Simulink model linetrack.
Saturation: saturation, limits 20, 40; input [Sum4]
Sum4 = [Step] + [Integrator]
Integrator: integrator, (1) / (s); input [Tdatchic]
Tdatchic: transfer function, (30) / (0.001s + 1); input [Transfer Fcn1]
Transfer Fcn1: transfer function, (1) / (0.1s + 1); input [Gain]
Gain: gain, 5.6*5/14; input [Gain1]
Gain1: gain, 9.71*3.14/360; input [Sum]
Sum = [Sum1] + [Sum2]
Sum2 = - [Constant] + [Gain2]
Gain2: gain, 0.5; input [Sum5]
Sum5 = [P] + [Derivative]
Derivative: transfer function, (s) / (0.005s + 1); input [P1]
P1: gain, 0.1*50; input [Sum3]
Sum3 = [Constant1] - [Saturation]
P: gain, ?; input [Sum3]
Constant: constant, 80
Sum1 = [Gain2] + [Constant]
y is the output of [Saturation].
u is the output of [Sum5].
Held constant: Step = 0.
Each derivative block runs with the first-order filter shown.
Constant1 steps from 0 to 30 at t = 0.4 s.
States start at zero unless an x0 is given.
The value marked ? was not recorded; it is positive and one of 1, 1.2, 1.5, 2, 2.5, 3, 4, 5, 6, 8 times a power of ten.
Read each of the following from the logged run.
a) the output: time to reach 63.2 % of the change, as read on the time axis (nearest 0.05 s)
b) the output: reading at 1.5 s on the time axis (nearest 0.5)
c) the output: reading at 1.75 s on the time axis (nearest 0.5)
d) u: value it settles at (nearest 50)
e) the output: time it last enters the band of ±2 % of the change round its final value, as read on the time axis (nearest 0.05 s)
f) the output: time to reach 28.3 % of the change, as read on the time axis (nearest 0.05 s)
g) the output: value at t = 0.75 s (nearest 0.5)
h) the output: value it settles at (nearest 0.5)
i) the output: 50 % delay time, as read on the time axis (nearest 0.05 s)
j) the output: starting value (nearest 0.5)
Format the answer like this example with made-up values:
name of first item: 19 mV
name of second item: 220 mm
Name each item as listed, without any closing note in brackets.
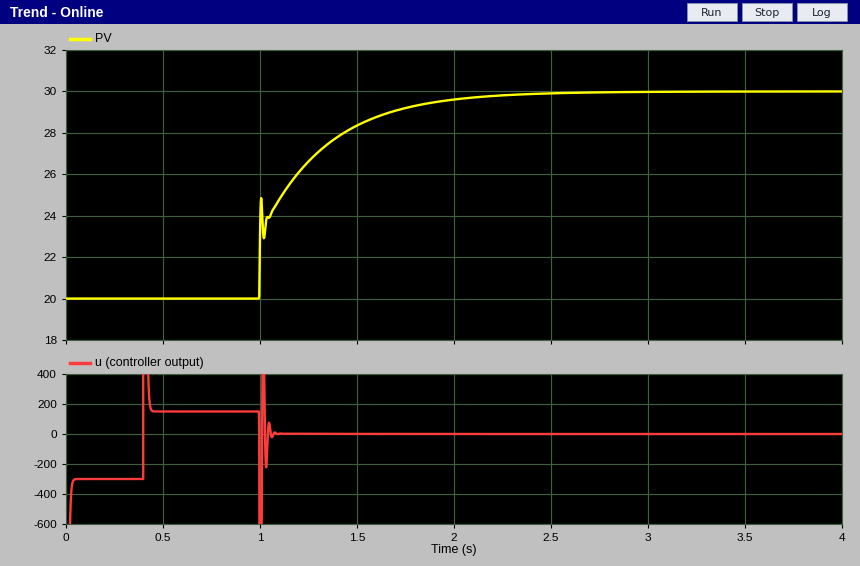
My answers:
the output: time to reach 63.2 % of the change, as read on the time axis: 1.20 s
the output: reading at 1.5 s on the time axis: 28.5
the output: reading at 1.75 s on the time axis: 29.0
u: value it settles at: 0
the output: time it last enters the band of ±2 % of the change round its final value, as read on the time axis: 2.25 s
the output: time to reach 28.3 % of the change, as read on the time axis: 1.00 s
the output: value at t = 0.75 s: 20.0
the output: value it settles at: 30.0
the output: 50 % delay time, as read on the time axis: 1.10 s
the output: starting value: 20.0
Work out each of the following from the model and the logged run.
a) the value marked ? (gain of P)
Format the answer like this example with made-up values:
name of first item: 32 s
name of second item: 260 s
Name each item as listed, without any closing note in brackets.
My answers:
the value marked ?: 15
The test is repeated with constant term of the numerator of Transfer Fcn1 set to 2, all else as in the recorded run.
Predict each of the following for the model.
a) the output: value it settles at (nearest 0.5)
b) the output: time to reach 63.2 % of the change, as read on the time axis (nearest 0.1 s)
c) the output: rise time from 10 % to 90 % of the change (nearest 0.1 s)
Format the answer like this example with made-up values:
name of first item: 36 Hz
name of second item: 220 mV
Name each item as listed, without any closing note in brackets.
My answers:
the output: value it settles at: 30.0
the output: time to reach 63.2 % of the change, as read on the time axis: 1.0 s
the output: rise time from 10 % to 90 % of the change: 0.7 s
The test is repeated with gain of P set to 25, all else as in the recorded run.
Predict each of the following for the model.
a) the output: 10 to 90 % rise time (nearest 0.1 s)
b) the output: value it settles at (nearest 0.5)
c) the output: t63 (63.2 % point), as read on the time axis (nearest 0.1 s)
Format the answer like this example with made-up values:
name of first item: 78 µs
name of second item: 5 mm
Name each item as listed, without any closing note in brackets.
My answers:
the output: 10 to 90 % rise time: 0.3 s
the output: value it settles at: 30.0
the output: t63 (63.2 % point), as read on the time axis: 1.1 s
